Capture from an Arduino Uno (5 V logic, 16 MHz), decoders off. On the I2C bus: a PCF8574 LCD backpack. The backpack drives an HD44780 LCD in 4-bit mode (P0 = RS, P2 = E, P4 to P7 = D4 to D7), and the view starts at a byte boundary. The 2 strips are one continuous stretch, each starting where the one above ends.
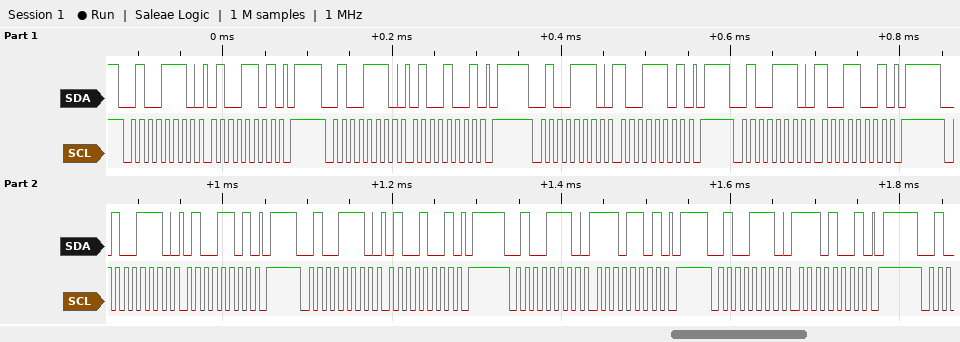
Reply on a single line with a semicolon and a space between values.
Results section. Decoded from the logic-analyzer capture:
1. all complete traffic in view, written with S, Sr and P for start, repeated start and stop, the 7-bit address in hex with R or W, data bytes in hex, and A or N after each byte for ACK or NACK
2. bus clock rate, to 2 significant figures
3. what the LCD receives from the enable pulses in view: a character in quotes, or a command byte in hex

S 27W A 4D A P S 27W A 49 A P S 27W A 9D A P S 27W A 99 A P S 27W A 4D A P S 27W A 49 A P S 27W A ED A P S 27W A E9 A P; 100 kHz; 'I' 'N'
